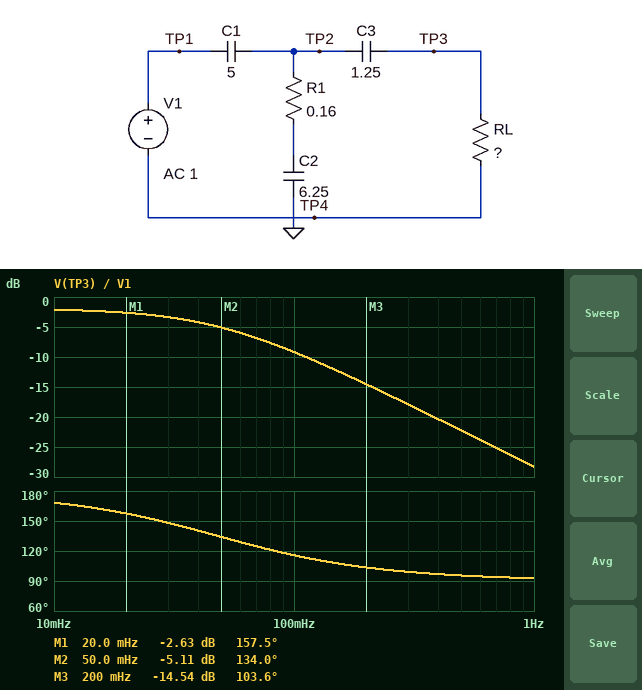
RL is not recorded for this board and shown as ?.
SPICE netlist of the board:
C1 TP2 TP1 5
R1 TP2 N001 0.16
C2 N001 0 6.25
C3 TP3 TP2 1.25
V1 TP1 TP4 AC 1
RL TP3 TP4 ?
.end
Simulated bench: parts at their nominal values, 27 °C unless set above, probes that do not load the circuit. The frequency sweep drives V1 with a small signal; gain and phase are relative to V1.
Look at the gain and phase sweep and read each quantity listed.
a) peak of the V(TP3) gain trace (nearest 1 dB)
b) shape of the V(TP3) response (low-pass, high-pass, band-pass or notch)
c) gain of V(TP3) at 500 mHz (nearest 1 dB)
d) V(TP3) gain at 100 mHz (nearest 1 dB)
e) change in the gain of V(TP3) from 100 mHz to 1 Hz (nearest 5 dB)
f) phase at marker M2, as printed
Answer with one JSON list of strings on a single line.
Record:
["-2 dB", "low-pass", "-22 dB", "-9 dB", "-20 dB", "134.0 deg"]
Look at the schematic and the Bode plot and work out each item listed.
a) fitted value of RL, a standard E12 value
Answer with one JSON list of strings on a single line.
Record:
["3.3 Ω"]
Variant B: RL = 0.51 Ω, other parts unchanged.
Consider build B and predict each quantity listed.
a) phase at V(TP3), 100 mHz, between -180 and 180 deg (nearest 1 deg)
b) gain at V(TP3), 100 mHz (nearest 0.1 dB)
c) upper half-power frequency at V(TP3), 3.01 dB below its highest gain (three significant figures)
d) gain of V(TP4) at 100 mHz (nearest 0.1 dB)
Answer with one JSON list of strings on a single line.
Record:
["162 deg", "-2.4 dB", "312 mHz", "-1.7 dB"]
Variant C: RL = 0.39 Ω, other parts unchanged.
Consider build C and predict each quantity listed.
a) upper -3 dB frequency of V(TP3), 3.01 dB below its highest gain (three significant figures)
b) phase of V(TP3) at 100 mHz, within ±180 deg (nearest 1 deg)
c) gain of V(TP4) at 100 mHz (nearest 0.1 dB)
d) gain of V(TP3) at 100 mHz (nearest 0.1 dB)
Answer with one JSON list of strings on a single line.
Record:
["408 mHz", "166 deg", "-1.8 dB", "-2.2 dB"]
